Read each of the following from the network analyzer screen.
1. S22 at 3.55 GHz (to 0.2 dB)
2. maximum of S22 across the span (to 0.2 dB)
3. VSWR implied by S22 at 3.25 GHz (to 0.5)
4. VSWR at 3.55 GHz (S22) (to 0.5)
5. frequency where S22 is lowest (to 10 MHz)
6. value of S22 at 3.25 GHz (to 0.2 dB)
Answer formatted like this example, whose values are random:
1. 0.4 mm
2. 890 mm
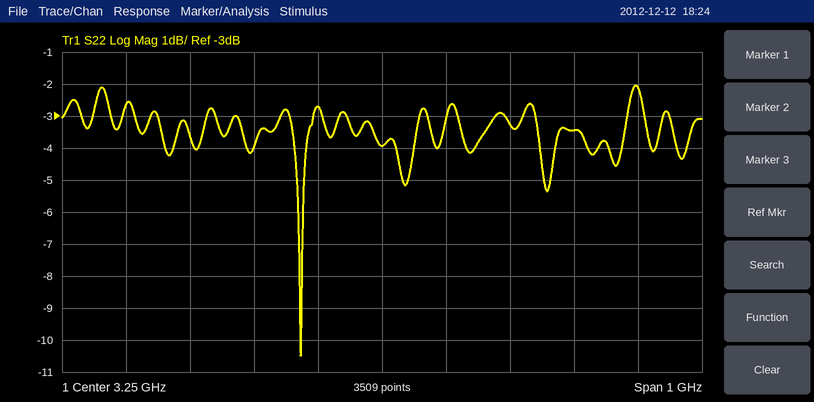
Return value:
1. -3.4 dB
2. -2.0 dB
3. 4.5
4. 5.0
5. 3.12 GHz
6. -4.0 dB
